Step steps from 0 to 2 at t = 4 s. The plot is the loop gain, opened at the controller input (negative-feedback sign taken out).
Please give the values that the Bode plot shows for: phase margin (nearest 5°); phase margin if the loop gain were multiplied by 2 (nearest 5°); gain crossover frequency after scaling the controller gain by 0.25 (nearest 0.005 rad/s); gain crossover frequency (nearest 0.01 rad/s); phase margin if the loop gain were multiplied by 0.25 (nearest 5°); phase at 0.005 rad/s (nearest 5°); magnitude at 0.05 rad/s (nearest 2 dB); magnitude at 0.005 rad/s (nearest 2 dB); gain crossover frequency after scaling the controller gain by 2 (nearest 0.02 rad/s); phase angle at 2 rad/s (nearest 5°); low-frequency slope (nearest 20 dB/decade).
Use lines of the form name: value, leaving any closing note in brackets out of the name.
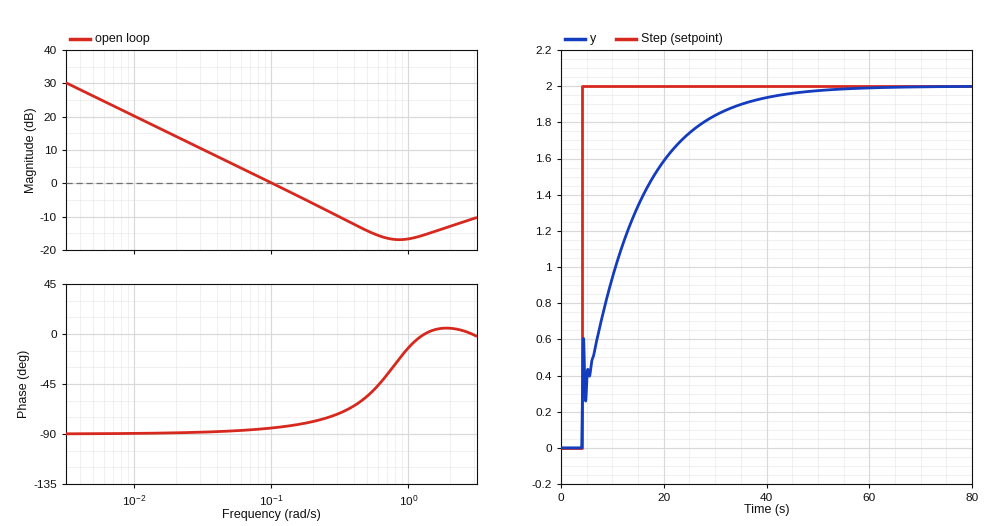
phase margin: 95°
phase margin if the loop gain were multiplied by 2: 100°
gain crossover frequency after scaling the controller gain by 0.25: 0.025 rad/s
gain crossover frequency: 0.10 rad/s
phase margin if the loop gain were multiplied by 0.25: 90°
phase at 0.005 rad/s: -90°
magnitude at 0.05 rad/s: 6 dB
magnitude at 0.005 rad/s: 26 dB
gain crossover frequency after scaling the controller gain by 2: 0.20 rad/s
phase angle at 2 rad/s: 5°
low-frequency slope: -20 dB/decade
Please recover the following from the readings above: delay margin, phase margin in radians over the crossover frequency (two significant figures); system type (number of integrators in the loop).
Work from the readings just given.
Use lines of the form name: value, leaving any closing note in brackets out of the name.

delay margin, phase margin in radians over the crossover frequency: 17 s
system type: 1
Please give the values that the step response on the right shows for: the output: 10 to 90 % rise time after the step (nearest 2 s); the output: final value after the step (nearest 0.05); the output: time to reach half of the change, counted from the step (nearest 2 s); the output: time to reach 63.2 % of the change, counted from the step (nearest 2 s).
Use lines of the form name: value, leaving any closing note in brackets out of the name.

the output: 10 to 90 % rise time after the step: 24 s
the output: final value after the step: 2.00
the output: time to reach half of the change, counted from the step: 6 s
the output: time to reach 63.2 % of the change, counted from the step: 10 s
